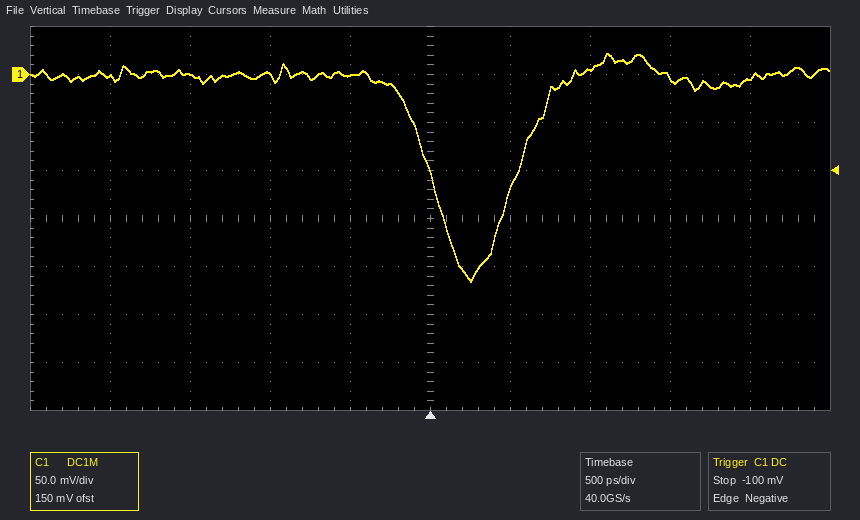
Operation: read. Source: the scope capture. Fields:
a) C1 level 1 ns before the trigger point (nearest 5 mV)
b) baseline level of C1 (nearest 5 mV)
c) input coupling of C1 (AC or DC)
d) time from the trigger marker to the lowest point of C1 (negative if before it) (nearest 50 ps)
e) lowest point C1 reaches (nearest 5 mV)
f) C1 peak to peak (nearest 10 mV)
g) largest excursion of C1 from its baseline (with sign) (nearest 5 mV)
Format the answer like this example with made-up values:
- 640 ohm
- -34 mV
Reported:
- 0 mV
- 0 mV
- DC
- +250 ps
- -215 mV
- 240 mV
- -215 mV
